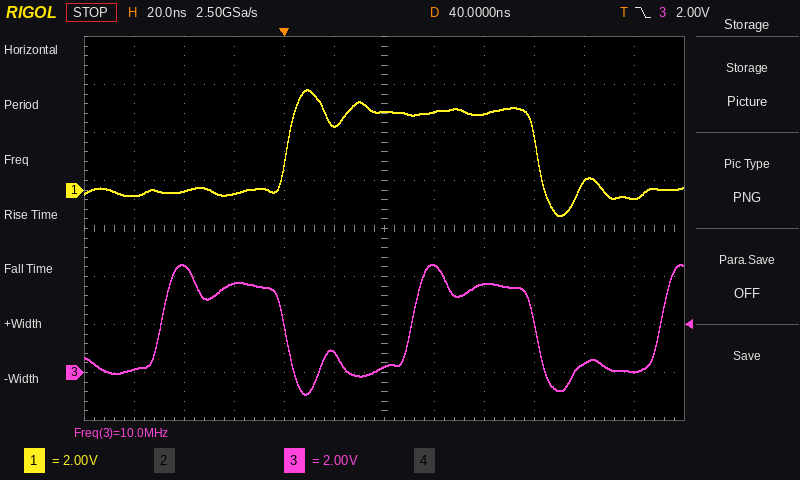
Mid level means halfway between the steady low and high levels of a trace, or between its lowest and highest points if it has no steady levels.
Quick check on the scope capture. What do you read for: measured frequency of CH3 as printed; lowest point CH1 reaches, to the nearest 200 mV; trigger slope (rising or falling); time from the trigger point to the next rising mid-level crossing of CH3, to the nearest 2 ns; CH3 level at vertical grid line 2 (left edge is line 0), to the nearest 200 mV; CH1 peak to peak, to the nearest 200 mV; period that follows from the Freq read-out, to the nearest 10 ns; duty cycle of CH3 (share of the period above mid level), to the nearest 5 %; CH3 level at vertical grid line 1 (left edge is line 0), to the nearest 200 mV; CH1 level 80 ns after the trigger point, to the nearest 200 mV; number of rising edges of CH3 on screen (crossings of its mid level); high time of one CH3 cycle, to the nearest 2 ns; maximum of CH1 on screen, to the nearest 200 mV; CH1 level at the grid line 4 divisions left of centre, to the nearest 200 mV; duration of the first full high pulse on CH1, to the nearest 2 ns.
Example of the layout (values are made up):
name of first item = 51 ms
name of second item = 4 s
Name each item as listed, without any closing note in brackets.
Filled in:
measured frequency of CH3 as printed = 10.0 MHz
lowest point CH1 reaches, to the nearest 200 mV = -1.0 V
trigger slope = falling
time from the trigger point to the next rising mid-level crossing of CH3, to the nearest 2 ns = 50 ns
CH3 level at vertical grid line 2 (left edge is line 0), to the nearest 200 mV = 4.4 V
CH1 peak to peak, to the nearest 200 mV = 5.2 V
period that follows from the Freq read-out, to the nearest 10 ns = 100 ns
duty cycle of CH3 (share of the period above mid level), to the nearest 5 % = 50 %
CH3 level at vertical grid line 1 (left edge is line 0), to the nearest 200 mV = 200 mV
CH1 level 80 ns after the trigger point, to the nearest 200 mV = 3.2 V
number of rising edges of CH3 on screen = 3
high time of one CH3 cycle, to the nearest 2 ns = 50 ns
maximum of CH1 on screen, to the nearest 200 mV = 4.2 V
CH1 level at the grid line 4 divisions left of centre, to the nearest 200 mV = 0.0 V
duration of the first full high pulse on CH1, to the nearest 2 ns = 100 ns
